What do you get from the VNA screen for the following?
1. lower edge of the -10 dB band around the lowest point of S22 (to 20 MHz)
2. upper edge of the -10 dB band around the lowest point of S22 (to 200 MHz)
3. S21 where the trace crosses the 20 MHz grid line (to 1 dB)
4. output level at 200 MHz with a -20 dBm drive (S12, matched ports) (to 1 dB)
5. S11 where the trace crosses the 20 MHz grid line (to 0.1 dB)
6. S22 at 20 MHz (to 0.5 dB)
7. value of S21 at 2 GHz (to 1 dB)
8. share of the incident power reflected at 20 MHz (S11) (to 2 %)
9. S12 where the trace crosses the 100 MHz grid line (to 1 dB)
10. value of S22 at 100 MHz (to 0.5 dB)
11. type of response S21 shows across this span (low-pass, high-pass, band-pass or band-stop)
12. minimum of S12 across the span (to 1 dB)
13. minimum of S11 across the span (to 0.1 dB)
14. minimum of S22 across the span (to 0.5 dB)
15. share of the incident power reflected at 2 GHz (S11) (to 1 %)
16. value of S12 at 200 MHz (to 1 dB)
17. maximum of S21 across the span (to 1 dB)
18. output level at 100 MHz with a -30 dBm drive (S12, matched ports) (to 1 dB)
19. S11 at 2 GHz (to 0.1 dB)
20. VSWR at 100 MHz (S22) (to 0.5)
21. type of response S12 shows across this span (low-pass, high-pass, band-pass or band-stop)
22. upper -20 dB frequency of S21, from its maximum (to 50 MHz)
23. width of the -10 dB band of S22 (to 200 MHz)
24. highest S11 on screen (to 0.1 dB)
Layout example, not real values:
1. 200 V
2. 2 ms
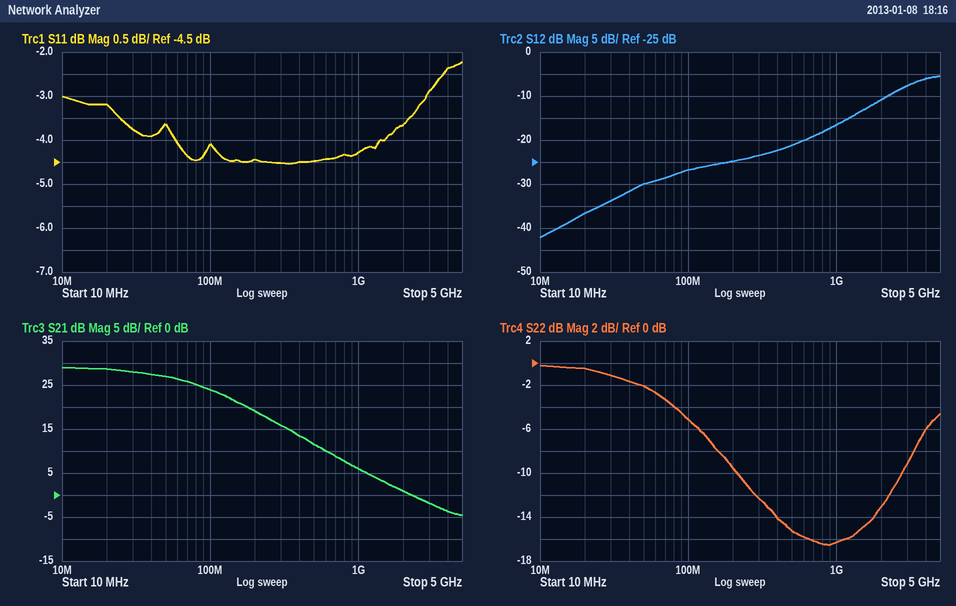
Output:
1. 220 MHz
2. 2.8 GHz
3. 29 dB
4. -45 dBm
5. -3.2 dB
6. -0.5 dB
7. 1 dB
8. 48 %
9. -27 dB
10. -5.0 dB
11. low-pass
12. -42 dB
13. -4.5 dB
14. -16.5 dB
15. 43 %
16. -25 dB
17. 29 dB
18. -57 dBm
19. -3.7 dB
20. 3.5
21. high-pass
22. 700 MHz
23. 2.6 GHz
24. -2.2 dB
